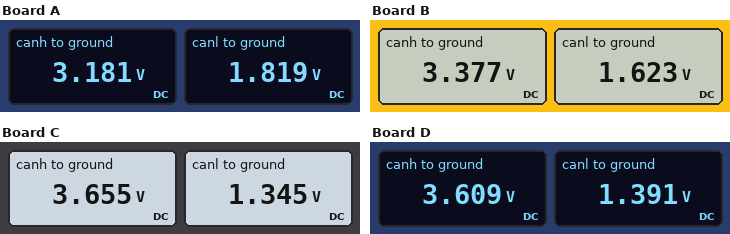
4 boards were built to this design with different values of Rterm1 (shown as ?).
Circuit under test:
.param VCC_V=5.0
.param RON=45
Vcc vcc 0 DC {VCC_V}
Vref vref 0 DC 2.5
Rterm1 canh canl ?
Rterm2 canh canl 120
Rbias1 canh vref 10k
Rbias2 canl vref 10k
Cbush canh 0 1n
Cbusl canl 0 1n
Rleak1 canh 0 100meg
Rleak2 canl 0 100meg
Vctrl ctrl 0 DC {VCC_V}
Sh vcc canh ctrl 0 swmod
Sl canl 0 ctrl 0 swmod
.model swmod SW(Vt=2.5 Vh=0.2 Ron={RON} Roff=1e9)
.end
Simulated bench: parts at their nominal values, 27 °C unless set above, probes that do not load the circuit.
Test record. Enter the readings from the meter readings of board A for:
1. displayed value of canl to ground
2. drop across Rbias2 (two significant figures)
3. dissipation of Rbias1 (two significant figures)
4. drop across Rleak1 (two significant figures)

1.819 V
680 mV
46 µW
3.2 V
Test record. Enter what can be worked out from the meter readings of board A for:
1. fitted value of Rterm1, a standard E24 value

47 Ω
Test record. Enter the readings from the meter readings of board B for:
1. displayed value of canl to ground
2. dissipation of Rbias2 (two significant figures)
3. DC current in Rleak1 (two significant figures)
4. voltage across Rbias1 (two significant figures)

1.623 V
77 µW
34 nA
880 mV
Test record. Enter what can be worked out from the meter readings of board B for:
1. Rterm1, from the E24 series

82 Ω
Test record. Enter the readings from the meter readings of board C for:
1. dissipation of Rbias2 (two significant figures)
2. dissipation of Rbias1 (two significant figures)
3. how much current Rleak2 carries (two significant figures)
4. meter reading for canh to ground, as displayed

130 µW
130 µW
13 nA
3.655 V
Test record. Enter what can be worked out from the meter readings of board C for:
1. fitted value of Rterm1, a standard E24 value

220 Ω
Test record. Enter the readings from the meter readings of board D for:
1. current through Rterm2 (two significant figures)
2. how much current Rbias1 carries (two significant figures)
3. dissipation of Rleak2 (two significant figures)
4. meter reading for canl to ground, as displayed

18 mA
110 µA
19 nW
1.391 V
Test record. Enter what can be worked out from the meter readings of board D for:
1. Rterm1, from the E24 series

180 Ω
